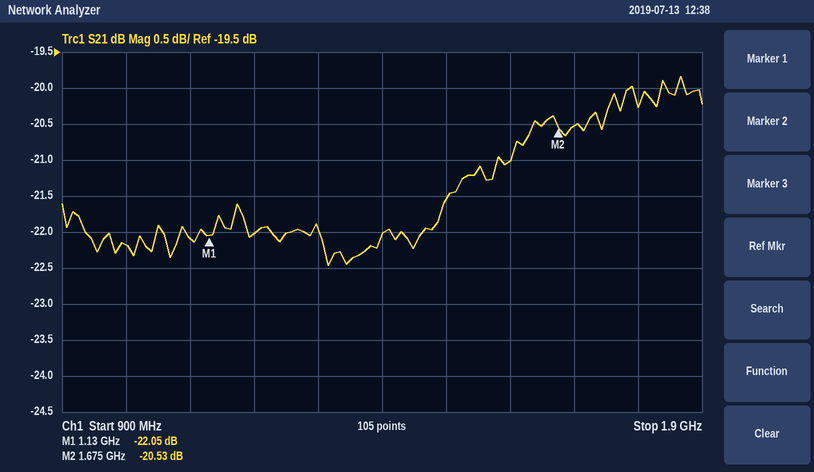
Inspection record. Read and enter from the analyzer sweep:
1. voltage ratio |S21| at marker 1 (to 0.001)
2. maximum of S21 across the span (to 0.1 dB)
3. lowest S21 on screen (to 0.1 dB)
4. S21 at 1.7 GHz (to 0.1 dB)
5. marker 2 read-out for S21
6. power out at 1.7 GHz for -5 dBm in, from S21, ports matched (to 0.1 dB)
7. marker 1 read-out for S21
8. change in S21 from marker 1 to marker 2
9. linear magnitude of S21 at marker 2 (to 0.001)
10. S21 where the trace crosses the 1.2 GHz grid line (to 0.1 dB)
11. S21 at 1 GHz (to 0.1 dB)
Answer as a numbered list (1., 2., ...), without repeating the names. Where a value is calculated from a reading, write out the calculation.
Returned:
1. 10^(-22.05/20) ≈ 0.079
2. -19.8 dB
3. -22.5 dB
4. -20.5 dB
5. -20.53 dB
6. -5 dBm + (-20.5 dB) = -25.5 dBm
7. -22.05 dB
8. -20.53 − (-22.05) = 1.52 dB
9. 10^(-20.53/20) ≈ 0.094
10. -22.0 dB
11. -22.2 dB
